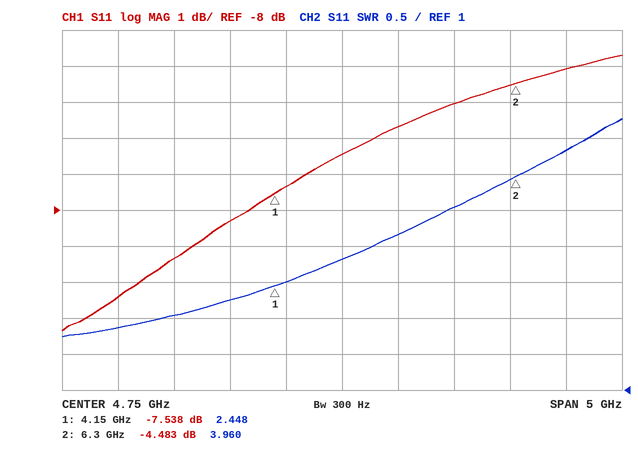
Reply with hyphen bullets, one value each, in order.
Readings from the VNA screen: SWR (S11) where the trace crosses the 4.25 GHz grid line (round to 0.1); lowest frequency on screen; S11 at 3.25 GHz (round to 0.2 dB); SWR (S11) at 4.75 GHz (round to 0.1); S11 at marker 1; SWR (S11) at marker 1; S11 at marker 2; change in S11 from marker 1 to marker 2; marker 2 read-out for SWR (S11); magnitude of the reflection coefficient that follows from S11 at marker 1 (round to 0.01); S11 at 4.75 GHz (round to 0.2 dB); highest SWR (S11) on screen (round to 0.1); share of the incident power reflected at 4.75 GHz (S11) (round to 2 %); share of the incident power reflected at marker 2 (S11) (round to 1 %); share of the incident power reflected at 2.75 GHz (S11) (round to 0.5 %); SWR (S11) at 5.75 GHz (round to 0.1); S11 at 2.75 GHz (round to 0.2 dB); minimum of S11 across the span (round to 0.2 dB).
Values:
- 2.5
- 2.25 GHz
- -9.4 dB
- 2.8
- -7.538 dB
- 2.448
- -4.483 dB
- 3.055 dB
- 3.960
- 0.42
- -6.4 dB
- 4.8
- 22 %
- 36 %
- 9.0 %
- 3.5
- -10.4 dB
- -11.4 dB
